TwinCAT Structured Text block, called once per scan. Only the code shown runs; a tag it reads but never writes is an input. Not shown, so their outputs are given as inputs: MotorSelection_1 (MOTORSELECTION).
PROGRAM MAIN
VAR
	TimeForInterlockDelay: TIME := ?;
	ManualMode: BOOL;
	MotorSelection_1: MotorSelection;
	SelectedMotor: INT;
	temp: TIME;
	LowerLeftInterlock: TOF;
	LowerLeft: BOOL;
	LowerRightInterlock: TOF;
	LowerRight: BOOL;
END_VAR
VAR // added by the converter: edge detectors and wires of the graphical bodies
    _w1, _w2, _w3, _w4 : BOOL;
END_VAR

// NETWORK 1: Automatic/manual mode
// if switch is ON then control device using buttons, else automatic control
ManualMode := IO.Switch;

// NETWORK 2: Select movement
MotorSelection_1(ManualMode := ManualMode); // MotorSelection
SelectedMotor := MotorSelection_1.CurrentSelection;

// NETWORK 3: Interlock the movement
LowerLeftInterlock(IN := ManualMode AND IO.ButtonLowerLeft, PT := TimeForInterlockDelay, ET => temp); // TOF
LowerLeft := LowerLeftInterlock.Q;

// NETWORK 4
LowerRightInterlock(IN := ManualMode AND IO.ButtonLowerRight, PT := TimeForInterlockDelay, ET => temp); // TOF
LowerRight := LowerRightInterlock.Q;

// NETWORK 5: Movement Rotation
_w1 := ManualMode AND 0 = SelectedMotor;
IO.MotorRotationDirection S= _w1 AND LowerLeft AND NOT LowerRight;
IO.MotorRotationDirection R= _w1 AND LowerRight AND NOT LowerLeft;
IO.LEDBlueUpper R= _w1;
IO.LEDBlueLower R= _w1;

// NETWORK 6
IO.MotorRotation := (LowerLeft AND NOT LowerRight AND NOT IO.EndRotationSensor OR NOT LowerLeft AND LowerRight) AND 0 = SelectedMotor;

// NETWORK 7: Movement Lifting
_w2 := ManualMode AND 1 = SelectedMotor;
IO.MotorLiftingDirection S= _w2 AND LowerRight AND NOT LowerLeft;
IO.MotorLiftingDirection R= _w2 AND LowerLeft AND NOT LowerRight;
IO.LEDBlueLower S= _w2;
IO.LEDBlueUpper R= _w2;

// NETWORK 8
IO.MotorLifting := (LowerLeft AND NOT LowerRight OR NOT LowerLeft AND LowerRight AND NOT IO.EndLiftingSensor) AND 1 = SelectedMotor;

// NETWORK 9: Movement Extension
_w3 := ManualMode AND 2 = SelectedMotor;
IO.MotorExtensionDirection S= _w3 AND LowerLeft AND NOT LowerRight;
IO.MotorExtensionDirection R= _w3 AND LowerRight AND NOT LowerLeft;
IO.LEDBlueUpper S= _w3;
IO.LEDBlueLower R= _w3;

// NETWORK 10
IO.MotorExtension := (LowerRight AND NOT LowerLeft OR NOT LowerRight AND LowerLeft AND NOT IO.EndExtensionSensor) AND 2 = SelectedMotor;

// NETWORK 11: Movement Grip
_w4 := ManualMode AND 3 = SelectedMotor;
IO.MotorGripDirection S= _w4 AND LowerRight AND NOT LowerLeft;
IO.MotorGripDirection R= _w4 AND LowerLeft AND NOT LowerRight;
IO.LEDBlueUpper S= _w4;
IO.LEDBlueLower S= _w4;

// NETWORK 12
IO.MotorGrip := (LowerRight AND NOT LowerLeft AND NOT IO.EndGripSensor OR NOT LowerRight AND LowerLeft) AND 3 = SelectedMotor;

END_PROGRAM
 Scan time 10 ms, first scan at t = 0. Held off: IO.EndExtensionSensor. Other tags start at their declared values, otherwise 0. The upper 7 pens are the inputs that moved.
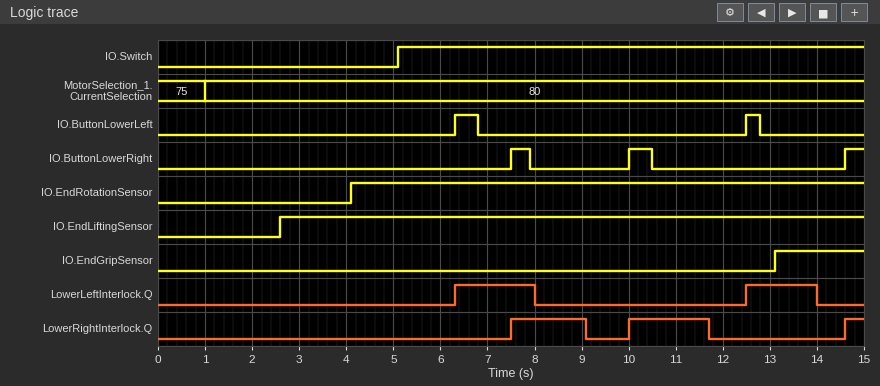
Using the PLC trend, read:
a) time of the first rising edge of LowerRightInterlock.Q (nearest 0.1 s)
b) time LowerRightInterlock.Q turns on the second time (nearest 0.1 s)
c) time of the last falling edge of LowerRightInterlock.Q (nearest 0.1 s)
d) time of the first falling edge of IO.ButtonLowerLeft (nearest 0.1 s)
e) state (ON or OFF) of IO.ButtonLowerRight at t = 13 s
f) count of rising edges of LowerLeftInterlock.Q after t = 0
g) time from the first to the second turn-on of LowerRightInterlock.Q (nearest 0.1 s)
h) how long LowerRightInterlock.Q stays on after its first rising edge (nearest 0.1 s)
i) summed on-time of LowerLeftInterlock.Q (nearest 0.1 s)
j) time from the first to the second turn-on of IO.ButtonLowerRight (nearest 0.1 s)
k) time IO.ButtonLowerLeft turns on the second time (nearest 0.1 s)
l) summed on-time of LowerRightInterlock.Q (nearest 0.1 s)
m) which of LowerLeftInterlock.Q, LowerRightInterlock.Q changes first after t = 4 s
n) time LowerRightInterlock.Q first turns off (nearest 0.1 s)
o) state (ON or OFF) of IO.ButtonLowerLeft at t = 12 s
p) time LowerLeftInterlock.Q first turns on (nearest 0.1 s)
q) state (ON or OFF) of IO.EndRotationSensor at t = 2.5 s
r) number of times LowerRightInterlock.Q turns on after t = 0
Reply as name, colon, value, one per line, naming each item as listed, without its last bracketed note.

time of the first rising edge of LowerRightInterlock.Q: 7.5 s
time LowerRightInterlock.Q turns on the second time: 10.0 s
time of the last falling edge of LowerRightInterlock.Q: 11.7 s
time of the first falling edge of IO.ButtonLowerLeft: 6.8 s
state (ON or OFF) of IO.ButtonLowerRight at t = 13 s: OFF
count of rising edges of LowerLeftInterlock.Q after t = 0: 2
time from the first to the second turn-on of LowerRightInterlock.Q: 2.5 s
how long LowerRightInterlock.Q stays on after its first rising edge: 1.6 s
summed on-time of LowerLeftInterlock.Q: 3.2 s
time from the first to the second turn-on of IO.ButtonLowerRight: 2.5 s
time IO.ButtonLowerLeft turns on the second time: 12.5 s
summed on-time of LowerRightInterlock.Q: 3.7 s
which of LowerLeftInterlock.Q, LowerRightInterlock.Q changes first after t = 4 s: LowerLeftInterlock.Q
time LowerRightInterlock.Q first turns off: 9.1 s
state (ON or OFF) of IO.ButtonLowerLeft at t = 12 s: OFF
time LowerLeftInterlock.Q first turns on: 6.3 s
state (ON or OFF) of IO.EndRotationSensor at t = 2.5 s: OFF
number of times LowerRightInterlock.Q turns on after t = 0: 3
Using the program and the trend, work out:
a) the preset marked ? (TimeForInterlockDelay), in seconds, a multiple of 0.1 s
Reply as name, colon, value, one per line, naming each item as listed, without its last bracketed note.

the preset marked ? (TimeForInterlockDelay), in seconds, a multiple of 0.1 s: 1.2 s
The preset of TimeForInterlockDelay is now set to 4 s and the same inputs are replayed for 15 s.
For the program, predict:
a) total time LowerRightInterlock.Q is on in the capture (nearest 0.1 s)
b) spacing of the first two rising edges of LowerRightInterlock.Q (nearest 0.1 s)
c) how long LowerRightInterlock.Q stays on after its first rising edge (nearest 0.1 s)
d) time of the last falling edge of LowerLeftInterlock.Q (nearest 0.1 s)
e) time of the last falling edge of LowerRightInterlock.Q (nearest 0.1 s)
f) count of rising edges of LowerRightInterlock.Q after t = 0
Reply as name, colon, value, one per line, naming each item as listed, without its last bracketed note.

total time LowerRightInterlock.Q is on in the capture: 7.4 s
spacing of the first two rising edges of LowerRightInterlock.Q: 7.1 s
how long LowerRightInterlock.Q stays on after its first rising edge: 7.0 s
time of the last falling edge of LowerLeftInterlock.Q: 10.8 s
time of the last falling edge of LowerRightInterlock.Q: 14.5 s
count of rising edges of LowerRightInterlock.Q after t = 0: 2
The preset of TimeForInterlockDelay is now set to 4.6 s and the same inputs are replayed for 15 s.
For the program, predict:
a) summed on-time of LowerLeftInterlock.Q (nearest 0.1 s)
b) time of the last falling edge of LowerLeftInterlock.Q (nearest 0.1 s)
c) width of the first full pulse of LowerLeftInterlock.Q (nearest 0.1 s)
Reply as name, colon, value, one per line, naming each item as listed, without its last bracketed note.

summed on-time of LowerLeftInterlock.Q: 7.6 s
time of the last falling edge of LowerLeftInterlock.Q: 11.4 s
width of the first full pulse of LowerLeftInterlock.Q: 5.1 s
